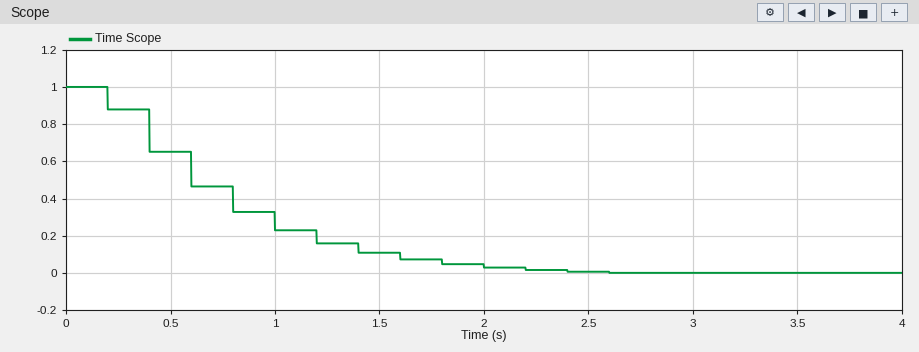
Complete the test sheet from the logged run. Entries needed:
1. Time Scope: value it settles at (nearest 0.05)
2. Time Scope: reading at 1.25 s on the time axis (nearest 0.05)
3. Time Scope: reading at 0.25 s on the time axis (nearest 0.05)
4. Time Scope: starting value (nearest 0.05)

0.00
0.15
0.90
1.00
